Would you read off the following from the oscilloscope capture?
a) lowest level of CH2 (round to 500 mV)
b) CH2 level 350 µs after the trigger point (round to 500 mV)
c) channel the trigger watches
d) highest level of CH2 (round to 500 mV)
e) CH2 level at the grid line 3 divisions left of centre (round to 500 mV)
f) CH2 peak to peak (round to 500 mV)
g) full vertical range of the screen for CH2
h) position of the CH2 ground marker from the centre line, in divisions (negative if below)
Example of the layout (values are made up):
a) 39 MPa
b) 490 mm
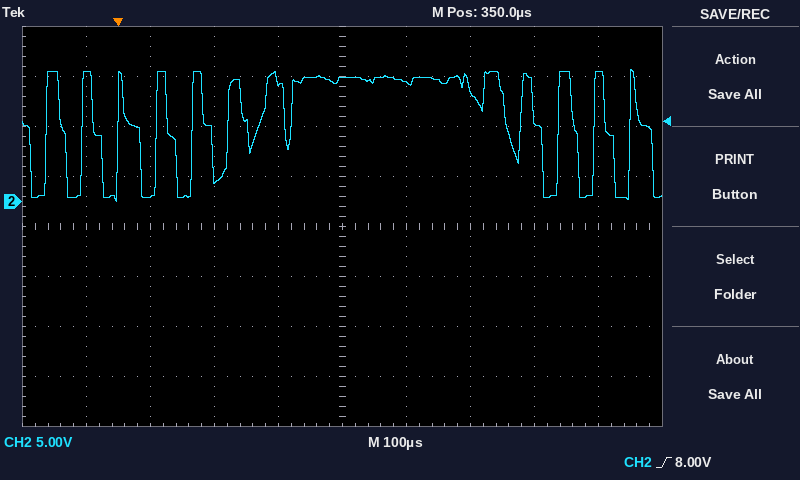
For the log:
a) 0.0 V
b) 12.5 V
c) CH2
d) 13.0 V
e) 500 mV
f) 13.0 V
g) 40 V
h) +0.5 div
